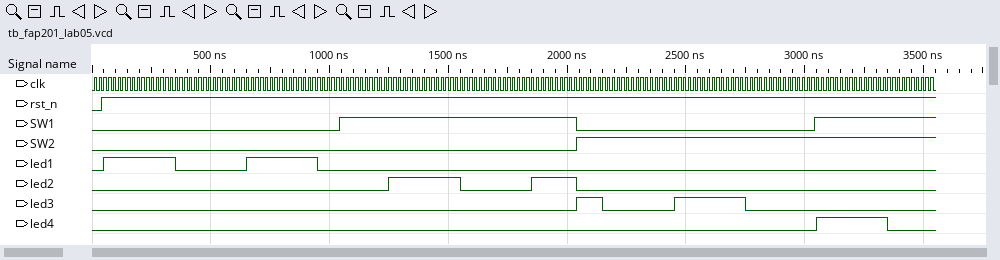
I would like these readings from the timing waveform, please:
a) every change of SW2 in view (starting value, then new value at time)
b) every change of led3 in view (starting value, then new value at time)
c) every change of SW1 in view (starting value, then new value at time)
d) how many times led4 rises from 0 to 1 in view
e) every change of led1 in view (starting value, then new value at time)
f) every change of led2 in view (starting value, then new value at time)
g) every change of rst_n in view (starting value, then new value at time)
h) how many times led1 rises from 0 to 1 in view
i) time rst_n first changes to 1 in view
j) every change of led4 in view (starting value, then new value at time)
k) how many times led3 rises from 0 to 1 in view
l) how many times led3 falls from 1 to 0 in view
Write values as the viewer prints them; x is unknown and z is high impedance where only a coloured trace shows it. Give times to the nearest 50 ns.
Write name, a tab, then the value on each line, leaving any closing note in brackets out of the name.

every change of SW2 in view	0, 1 at 2050 ns
every change of led3 in view	0, 1 at 2050 ns, 0 at 2150 ns, 1 at 2450 ns, 0 at 2750 ns
every change of SW1 in view	0, 1 at 1050 ns, 0 at 2050 ns, 1 at 3050 ns
how many times led4 rises from 0 to 1 in view	1
every change of led1 in view	0, 1 at 50 ns, 0 at 350 ns, 1 at 650 ns, 0 at 950 ns
every change of led2 in view	0, 1 at 1250 ns, 0 at 1550 ns, 1 at 1850 ns, 0 at 2050 ns
every change of rst_n in view	0, 1 at 50 ns
how many times led1 rises from 0 to 1 in view	2
time rst_n first changes to 1 in view	50 ns
every change of led4 in view	0, 1 at 3050 ns, 0 at 3350 ns
how many times led3 rises from 0 to 1 in view	2
how many times led3 falls from 1 to 0 in view	2
